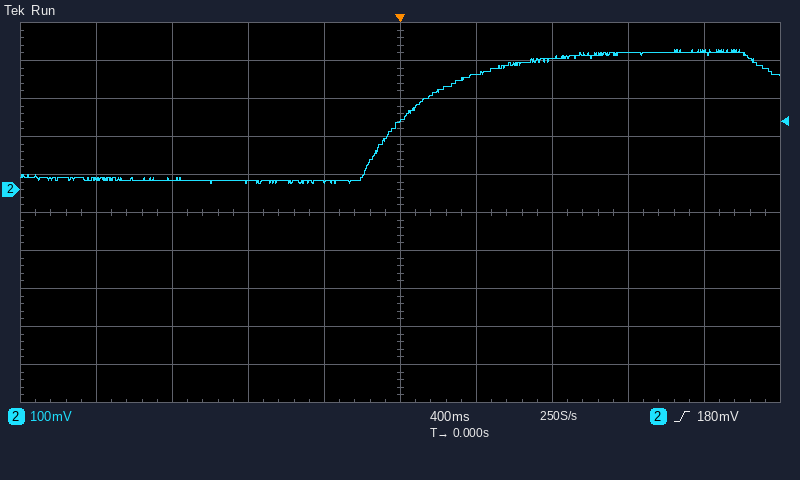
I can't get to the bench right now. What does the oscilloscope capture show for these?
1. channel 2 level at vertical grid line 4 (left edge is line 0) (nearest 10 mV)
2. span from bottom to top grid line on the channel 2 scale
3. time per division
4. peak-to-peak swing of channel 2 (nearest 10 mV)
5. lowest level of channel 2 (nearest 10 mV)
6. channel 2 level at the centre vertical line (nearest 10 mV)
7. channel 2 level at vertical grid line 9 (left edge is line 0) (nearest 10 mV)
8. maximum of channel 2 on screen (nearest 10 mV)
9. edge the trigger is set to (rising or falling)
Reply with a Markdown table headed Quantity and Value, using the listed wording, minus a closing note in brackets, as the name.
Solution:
| Quantity | Value |
|---|---|
| channel 2 level at vertical grid line 4 (left edge is line 0) | 20 mV |
| span from bottom to top grid line on the channel 2 scale | 1 V |
| time per division | 400 ms |
| peak-to-peak swing of channel 2 | 350 mV |
| lowest level of channel 2 | 20 mV |
| channel 2 level at the centre vertical line | 180 mV |
| channel 2 level at vertical grid line 9 (left edge is line 0) | 360 mV |
| maximum of channel 2 on screen | 370 mV |
| edge the trigger is set to | rising |
